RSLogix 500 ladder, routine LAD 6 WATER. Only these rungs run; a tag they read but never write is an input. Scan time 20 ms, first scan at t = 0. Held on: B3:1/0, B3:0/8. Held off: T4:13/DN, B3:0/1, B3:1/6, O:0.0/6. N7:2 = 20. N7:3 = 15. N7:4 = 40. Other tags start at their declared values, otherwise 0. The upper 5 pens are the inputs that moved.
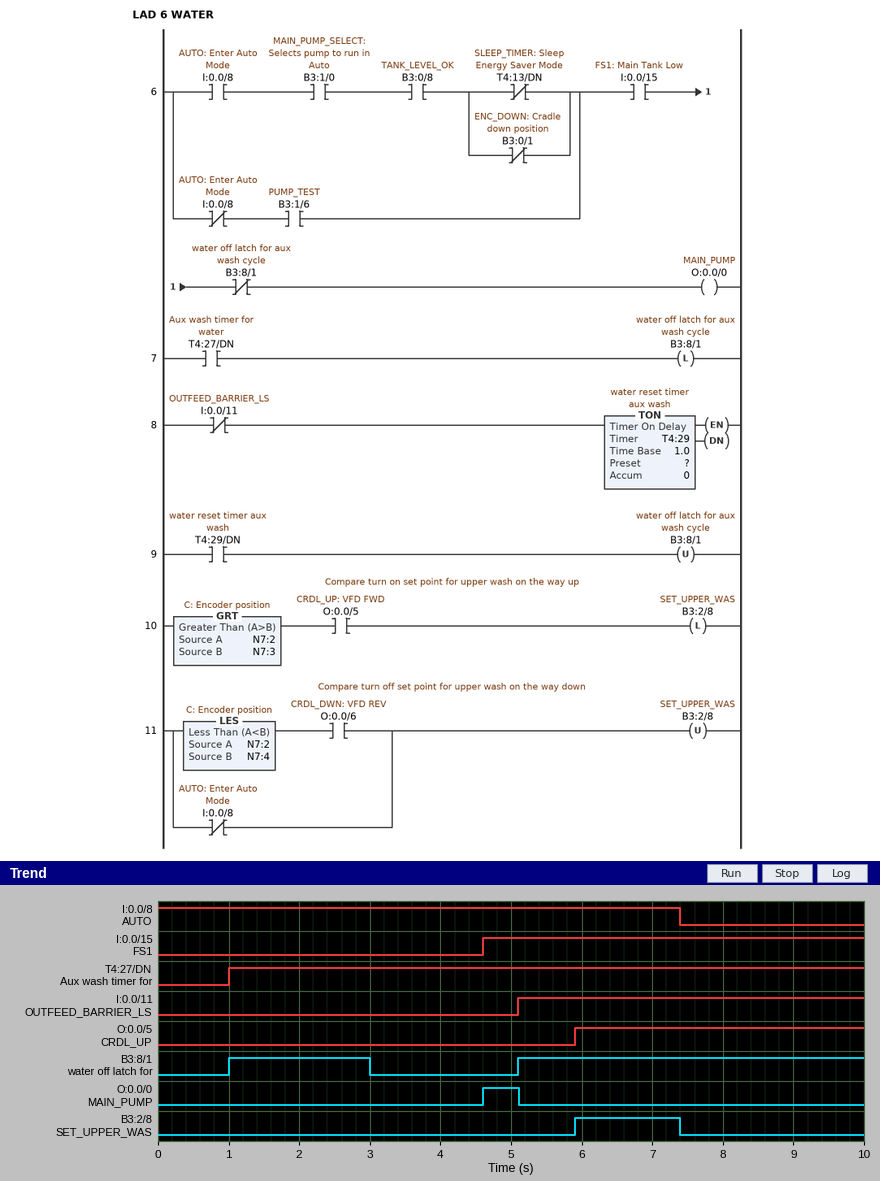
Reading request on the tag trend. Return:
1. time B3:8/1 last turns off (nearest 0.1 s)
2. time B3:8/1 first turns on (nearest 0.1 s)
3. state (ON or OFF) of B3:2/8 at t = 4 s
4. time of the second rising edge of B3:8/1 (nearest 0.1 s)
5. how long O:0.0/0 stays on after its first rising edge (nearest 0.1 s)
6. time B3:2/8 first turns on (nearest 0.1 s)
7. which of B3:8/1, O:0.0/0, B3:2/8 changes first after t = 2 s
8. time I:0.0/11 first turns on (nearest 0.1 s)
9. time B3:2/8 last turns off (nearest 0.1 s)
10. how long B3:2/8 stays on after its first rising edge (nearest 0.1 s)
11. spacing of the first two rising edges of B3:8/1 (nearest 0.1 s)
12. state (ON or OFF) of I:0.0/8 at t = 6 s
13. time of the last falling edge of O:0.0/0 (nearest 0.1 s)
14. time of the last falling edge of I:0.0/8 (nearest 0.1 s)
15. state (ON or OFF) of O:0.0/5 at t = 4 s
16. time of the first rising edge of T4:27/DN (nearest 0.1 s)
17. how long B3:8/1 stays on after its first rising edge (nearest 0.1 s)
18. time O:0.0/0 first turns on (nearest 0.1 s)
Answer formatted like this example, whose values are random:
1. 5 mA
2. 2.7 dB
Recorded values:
1. 3.0 s
2. 1.0 s
3. OFF
4. 5.1 s
5. 0.5 s
6. 5.9 s
7. B3:8/1
8. 5.1 s
9. 7.4 s
10. 1.5 s
11. 4.1 s
12. ON
13. 5.1 s
14. 7.4 s
15. OFF
16. 1.0 s
17. 2.0 s
18. 4.6 s
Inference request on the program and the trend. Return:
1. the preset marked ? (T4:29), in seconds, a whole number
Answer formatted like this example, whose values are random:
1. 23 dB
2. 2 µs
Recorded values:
1. 3 s
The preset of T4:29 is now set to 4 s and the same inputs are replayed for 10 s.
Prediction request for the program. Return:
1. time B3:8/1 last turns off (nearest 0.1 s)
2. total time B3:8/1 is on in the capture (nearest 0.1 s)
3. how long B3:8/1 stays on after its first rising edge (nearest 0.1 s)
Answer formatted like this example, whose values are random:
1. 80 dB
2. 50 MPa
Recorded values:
1. 4.0 s
2. 7.9 s
3. 3.0 s
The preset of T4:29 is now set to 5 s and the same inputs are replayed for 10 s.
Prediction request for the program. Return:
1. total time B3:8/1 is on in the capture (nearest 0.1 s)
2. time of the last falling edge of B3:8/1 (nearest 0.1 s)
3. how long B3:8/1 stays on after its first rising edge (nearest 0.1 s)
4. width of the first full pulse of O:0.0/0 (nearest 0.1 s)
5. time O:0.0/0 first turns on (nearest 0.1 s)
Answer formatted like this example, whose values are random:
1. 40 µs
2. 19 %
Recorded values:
1. 8.9 s
2. 5.0 s
3. 4.0 s
4. 0.1 s
5. 5.0 s
